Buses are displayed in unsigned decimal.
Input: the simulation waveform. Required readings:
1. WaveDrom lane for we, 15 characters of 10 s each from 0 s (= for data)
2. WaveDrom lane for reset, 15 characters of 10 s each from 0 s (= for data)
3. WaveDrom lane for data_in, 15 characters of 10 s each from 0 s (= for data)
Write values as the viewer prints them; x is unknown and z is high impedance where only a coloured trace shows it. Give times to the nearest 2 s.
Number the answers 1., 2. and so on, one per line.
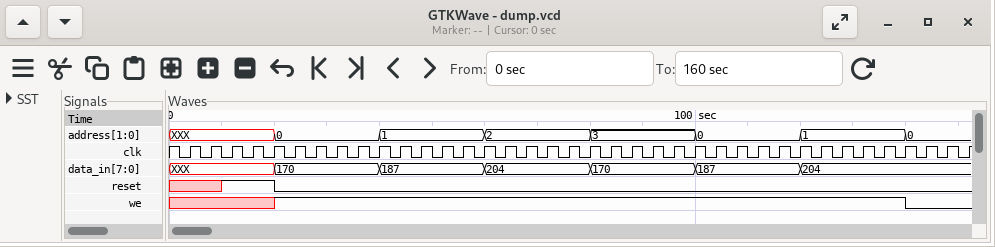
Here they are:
1. {name: 'we', wave: 'x.1...........0'}
2. {name: 'reset', wave: 'x10............'}
3. {name: 'data_in', wave: 'x.=.=.=.=.=.=..', data: '170 187 204 170 187 204'}
